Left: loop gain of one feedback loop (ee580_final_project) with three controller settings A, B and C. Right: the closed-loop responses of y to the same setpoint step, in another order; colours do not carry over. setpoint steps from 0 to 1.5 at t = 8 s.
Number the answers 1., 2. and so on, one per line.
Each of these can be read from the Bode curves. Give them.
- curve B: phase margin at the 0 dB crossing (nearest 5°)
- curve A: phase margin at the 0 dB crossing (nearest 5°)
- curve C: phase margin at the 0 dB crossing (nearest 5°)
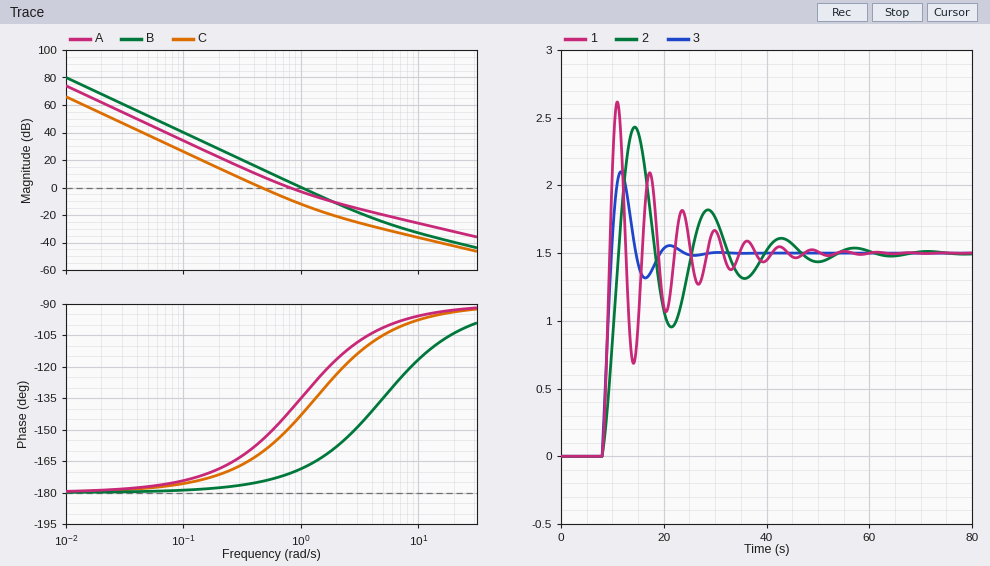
1. 10°
2. 40°
3. 20°
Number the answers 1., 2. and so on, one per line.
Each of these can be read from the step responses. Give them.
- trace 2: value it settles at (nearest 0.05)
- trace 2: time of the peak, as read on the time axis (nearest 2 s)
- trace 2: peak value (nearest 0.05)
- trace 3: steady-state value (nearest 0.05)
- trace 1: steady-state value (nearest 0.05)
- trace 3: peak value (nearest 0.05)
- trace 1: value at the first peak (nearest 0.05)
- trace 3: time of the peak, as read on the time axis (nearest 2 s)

1. 1.50
2. 14 s
3. 2.45
4. 1.50
5. 1.50
6. 2.10
7. 2.60
8. 12 s
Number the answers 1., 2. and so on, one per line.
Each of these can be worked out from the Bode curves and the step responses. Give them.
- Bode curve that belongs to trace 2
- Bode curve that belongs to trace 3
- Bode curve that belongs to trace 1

1. C
2. A
3. B
